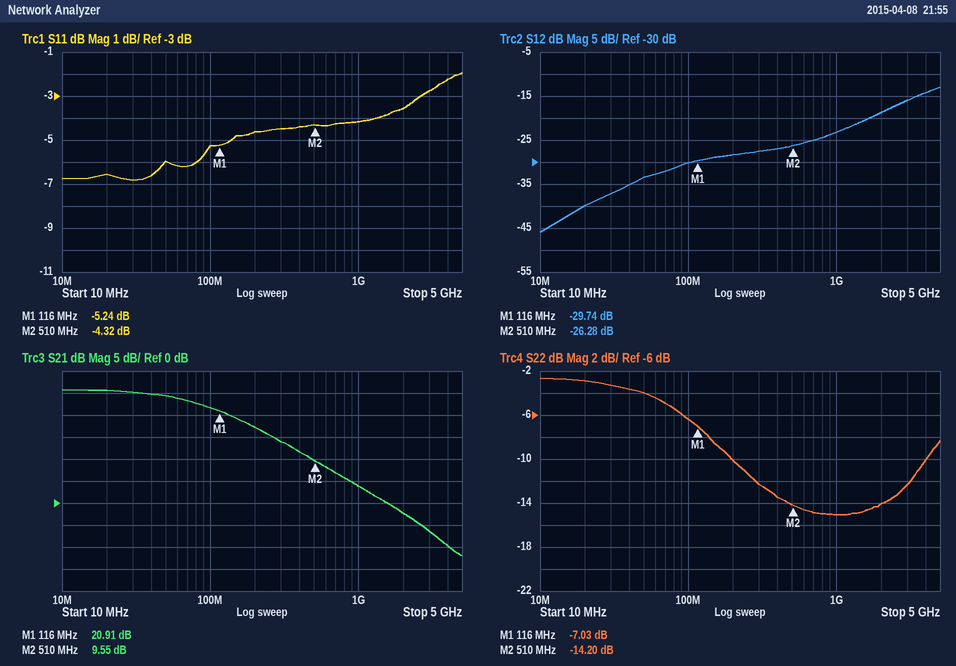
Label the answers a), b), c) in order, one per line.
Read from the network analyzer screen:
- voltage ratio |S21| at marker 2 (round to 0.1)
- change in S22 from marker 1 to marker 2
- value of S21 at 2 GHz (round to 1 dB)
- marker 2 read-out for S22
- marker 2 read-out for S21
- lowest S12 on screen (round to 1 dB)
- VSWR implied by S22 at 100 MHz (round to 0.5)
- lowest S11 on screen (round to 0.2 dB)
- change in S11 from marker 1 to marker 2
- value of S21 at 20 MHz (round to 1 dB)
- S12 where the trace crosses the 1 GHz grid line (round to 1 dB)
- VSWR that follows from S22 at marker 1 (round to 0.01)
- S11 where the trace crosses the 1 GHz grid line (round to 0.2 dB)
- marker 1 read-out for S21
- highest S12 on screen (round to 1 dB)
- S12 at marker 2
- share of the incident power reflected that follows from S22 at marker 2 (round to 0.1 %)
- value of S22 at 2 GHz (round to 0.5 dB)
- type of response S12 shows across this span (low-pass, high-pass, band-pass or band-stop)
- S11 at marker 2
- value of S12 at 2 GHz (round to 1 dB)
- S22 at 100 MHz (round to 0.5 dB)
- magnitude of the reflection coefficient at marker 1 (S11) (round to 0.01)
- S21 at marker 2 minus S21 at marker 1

a) 3.0
b) -7.17 dB
c) -2 dB
d) -14.20 dB
e) 9.55 dB
f) -46 dB
g) 3.0
h) -6.8 dB
i) 0.92 dB
j) 26 dB
k) -23 dB
l) 2.60
m) -4.2 dB
n) 20.91 dB
o) -13 dB
p) -26.28 dB
q) 3.8 %
r) -14.0 dB
s) high-pass
t) -4.32 dB
u) -19 dB
v) -6.5 dB
w) 0.55
x) -11.36 dB
